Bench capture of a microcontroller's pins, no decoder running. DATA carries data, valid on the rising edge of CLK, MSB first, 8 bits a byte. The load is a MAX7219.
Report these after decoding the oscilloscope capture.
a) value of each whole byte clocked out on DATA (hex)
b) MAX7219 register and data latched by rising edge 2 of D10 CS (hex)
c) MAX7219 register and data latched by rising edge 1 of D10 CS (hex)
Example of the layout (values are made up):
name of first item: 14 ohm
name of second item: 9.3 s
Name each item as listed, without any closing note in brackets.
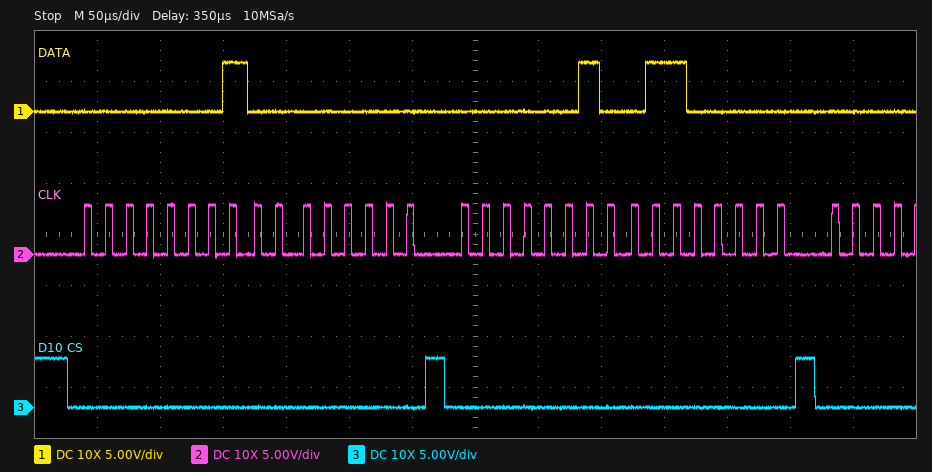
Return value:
value of each whole byte clocked out on DATA: 0x01 0x00 0x02 0x60
MAX7219 register and data latched by rising edge 2 of D10 CS: register 0x2, data 0x60
MAX7219 register and data latched by rising edge 1 of D10 CS: register 0x1, data 0x00
